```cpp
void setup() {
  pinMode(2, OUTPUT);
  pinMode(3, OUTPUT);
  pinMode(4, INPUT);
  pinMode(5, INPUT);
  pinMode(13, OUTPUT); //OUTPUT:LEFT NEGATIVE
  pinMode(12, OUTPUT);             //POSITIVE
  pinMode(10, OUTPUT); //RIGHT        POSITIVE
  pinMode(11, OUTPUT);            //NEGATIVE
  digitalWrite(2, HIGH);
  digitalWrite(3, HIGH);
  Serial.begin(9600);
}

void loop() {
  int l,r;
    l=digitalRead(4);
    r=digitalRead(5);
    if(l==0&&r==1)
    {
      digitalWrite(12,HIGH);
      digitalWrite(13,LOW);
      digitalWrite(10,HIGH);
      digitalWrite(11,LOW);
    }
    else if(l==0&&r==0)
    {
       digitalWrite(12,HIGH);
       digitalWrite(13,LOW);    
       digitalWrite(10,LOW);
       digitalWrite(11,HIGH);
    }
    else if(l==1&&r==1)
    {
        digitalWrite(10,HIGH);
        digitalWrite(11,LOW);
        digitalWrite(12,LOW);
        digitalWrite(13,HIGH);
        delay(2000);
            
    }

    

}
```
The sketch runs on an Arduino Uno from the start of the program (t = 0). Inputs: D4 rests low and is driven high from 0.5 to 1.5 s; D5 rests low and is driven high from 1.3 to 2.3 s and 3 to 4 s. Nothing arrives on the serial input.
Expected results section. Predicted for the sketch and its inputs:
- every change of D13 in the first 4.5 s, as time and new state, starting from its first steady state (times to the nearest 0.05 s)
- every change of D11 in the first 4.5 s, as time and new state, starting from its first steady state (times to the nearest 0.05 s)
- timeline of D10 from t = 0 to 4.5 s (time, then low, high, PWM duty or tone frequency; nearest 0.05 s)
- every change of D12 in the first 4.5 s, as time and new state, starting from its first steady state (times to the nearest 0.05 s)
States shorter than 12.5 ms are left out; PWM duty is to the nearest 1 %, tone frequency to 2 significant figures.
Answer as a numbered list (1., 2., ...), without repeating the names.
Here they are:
1. 0 s low; 1.3 s high; 3.3 s low
2. 0 s high; 1.3 s low; 4 s high
3. 0 s low; 1.3 s high; 4 s low
4. 0 s high; 1.3 s low; 3.3 s high
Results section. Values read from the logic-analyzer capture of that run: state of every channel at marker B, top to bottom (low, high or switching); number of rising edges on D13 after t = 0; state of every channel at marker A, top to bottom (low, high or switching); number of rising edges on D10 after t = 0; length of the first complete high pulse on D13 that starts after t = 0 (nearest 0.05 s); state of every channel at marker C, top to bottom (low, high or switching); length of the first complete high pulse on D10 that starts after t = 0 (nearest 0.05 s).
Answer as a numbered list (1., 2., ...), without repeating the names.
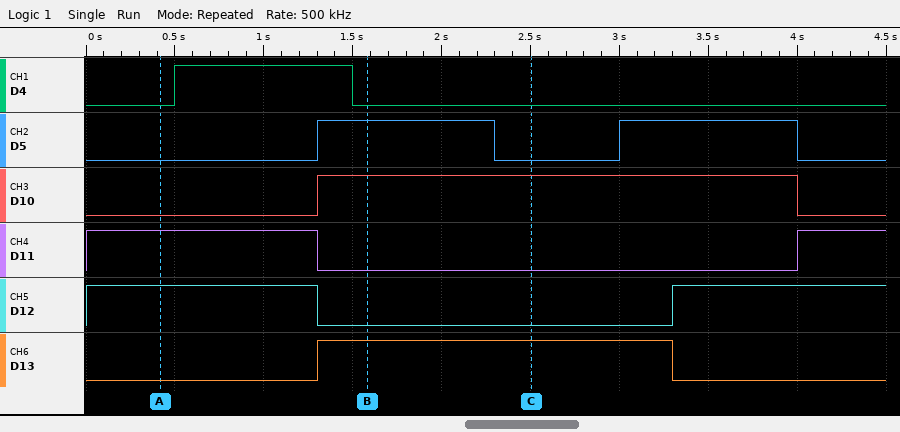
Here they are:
1. D4 low, D5 high, D10 high, D11 low, D12 low, D13 high
2. 1
3. D4 low, D5 low, D10 low, D11 high, D12 high, D13 low
4. 1
5. 2.00 s
6. D4 low, D5 low, D10 high, D11 low, D12 low, D13 high
7. 2.70 s
